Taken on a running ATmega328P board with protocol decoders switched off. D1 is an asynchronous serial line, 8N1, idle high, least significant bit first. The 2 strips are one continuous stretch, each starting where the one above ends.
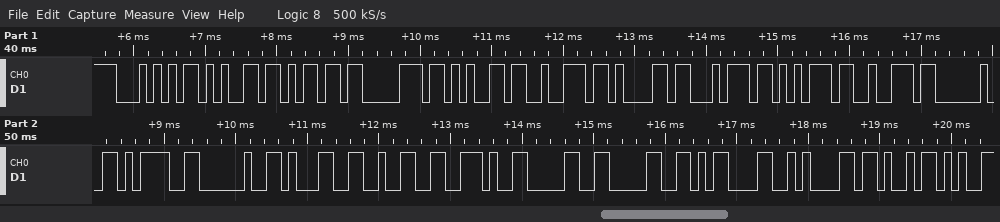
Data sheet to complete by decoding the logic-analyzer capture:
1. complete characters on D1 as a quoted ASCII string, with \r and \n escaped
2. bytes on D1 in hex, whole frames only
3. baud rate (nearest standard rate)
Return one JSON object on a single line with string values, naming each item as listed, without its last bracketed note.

{"complete characters on D1 as a quoted ASCII string, with \\r and \\n escaped": "\"Temperatur = 12.00\\r\\nK\"", "bytes on D1 in hex, whole frames only": "54 65 6D 70 65 72 61 74 75 72 20 3D 20 31 32 2E 30 30 0D 0A 4B", "baud rate": "9600 baud"}
